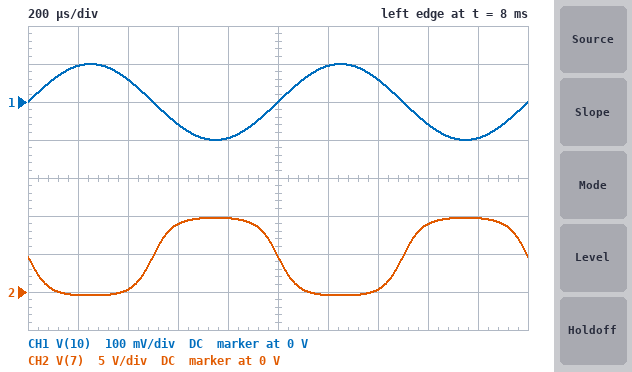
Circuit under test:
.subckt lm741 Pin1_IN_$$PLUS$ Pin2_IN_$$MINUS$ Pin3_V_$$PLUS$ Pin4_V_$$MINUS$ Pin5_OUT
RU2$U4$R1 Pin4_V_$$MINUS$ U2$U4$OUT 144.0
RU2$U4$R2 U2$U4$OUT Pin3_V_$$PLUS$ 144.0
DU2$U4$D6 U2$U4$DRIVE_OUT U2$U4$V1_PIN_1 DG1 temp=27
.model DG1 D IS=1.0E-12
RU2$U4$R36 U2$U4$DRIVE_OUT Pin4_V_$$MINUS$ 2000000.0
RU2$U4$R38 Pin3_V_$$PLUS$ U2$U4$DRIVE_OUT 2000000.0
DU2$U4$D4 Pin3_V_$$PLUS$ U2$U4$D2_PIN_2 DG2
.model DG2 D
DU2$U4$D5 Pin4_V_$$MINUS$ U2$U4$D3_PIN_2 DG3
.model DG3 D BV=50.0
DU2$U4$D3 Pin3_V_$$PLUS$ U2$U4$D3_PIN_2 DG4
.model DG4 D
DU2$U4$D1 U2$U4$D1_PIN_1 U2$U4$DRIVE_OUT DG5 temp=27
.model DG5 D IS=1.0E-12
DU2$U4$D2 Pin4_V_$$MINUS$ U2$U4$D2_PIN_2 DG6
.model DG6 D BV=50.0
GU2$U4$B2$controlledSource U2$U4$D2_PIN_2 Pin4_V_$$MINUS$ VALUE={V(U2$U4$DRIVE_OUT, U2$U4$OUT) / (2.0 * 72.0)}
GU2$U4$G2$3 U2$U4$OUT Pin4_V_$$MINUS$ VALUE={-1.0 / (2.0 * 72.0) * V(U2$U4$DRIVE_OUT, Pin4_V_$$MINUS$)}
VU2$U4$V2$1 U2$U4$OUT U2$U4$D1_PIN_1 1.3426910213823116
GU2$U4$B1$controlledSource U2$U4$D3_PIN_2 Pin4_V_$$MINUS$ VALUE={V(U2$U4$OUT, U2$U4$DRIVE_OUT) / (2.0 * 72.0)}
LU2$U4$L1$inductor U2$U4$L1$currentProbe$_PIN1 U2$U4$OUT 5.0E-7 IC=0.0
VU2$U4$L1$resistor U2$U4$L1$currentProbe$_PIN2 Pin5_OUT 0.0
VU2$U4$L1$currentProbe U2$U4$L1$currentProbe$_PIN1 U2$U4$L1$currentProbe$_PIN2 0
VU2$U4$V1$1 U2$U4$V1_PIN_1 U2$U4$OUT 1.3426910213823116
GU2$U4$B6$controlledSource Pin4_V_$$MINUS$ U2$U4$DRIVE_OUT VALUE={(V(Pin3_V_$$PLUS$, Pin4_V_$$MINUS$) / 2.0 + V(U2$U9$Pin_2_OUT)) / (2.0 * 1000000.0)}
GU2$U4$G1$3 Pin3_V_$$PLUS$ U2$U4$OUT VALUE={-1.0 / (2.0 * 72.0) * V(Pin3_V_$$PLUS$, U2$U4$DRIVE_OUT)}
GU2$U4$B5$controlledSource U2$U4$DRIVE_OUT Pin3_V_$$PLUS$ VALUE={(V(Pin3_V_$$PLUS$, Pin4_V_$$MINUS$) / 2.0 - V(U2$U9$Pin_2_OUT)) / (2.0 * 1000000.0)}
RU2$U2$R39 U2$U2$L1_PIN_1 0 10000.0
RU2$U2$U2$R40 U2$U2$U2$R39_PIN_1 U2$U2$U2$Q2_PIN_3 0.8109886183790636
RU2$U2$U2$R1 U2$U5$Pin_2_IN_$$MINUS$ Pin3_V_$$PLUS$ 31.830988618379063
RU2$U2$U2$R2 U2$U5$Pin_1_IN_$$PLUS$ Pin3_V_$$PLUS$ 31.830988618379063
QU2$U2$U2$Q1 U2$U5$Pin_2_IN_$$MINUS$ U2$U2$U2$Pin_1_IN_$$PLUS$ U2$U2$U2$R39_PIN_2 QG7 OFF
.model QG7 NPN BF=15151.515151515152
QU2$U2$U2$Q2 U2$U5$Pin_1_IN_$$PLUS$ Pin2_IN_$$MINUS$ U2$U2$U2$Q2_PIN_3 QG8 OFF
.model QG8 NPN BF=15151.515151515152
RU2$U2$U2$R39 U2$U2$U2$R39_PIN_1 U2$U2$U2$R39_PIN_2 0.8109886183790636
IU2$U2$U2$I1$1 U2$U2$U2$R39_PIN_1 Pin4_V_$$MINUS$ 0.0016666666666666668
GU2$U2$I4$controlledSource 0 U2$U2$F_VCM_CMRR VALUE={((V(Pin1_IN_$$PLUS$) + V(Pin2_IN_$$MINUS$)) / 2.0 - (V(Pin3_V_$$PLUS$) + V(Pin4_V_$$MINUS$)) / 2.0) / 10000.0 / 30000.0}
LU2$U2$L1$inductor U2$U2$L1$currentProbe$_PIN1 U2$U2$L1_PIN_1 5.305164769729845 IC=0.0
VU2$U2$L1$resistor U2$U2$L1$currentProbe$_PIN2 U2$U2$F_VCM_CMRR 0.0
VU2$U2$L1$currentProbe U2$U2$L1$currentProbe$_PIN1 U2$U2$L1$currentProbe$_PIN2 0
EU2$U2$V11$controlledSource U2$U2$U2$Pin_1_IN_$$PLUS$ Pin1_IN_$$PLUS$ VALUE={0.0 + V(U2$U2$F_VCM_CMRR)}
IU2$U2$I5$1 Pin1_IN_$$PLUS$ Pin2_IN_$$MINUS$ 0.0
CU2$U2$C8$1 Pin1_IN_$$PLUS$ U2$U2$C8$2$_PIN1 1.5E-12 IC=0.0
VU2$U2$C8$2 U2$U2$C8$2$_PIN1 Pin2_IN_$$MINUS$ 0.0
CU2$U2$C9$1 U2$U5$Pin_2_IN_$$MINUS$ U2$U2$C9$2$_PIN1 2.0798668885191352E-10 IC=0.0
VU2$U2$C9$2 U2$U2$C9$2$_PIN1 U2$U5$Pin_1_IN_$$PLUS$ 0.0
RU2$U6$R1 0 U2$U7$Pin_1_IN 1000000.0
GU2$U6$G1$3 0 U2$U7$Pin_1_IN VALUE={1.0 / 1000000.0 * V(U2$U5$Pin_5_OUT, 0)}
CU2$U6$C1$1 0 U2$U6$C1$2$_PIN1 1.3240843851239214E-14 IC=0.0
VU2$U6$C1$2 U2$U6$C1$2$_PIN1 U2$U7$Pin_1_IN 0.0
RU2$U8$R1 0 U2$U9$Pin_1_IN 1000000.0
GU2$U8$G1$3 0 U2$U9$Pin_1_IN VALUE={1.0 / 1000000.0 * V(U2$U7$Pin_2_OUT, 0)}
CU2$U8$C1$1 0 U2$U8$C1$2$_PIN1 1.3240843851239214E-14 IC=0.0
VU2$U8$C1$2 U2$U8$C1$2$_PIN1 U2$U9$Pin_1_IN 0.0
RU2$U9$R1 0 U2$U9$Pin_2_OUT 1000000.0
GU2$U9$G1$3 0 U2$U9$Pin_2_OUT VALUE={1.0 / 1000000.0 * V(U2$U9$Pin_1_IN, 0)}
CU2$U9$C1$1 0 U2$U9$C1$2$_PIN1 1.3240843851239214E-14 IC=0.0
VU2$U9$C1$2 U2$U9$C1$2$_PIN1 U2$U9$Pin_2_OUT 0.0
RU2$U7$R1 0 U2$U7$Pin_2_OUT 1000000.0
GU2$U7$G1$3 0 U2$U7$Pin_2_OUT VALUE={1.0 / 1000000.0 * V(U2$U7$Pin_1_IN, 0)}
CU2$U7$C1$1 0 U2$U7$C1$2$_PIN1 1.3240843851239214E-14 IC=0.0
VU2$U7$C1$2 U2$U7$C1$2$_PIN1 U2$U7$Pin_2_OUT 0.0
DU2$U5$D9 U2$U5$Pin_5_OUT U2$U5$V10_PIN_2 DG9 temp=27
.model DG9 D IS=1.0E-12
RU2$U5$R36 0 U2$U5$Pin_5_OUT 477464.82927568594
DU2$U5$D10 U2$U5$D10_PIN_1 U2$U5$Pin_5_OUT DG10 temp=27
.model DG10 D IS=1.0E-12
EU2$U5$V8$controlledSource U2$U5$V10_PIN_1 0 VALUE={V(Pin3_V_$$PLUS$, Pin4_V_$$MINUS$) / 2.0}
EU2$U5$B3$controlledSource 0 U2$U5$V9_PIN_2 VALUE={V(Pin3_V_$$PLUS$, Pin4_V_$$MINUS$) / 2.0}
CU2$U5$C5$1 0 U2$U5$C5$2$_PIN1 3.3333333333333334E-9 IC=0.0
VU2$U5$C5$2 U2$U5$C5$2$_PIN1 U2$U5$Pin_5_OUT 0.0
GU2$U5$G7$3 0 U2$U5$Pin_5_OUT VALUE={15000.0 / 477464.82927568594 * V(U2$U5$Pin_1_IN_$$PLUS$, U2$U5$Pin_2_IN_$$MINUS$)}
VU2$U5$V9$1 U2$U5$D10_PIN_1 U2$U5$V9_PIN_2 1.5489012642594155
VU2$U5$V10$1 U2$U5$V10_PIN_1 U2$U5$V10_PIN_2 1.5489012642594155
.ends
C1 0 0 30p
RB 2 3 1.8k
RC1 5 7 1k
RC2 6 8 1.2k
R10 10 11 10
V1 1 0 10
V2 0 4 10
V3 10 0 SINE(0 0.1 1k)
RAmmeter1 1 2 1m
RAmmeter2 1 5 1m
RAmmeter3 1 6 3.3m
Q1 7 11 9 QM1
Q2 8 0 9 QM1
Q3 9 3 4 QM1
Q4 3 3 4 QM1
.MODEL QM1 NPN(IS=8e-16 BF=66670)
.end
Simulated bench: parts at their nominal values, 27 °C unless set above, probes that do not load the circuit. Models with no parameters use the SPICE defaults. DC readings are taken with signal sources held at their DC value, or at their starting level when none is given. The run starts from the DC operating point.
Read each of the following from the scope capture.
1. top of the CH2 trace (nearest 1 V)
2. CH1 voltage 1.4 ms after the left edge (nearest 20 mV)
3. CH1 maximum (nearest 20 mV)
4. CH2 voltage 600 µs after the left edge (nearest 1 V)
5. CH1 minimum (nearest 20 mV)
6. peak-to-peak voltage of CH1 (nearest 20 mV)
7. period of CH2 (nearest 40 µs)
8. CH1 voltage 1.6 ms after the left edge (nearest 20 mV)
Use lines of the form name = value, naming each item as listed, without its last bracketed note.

top of the CH2 trace = 10 V
CH1 voltage 1.4 ms after the left edge = 60 mV
CH1 maximum = 100 mV
CH2 voltage 600 µs after the left edge = 9 V
CH1 minimum = -100 mV
peak-to-peak voltage of CH1 = 200 mV
period of CH2 = 1.00 ms
CH1 voltage 1.6 ms after the left edge = -60 mV
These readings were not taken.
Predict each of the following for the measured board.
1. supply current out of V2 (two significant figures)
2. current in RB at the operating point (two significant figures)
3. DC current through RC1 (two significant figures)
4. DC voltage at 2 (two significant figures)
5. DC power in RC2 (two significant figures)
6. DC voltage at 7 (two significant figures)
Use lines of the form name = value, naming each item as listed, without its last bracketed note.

supply current out of V2 = 21 mA
current in RB at the operating point = 11 mA
DC current through RC1 = 5.3 mA
DC voltage at 2 = 10 V
DC power in RC2 = 34 mW
DC voltage at 7 = 4.7 V
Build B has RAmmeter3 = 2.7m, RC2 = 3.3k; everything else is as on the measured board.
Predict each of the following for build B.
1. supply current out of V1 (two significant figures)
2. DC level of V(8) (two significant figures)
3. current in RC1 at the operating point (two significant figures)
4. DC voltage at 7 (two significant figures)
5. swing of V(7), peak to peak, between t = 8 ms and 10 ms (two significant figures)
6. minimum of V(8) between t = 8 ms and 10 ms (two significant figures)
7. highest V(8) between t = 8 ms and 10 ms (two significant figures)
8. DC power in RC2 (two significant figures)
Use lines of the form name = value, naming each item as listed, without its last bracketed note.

supply current out of V1 = 20 mA
DC level of V(8) = -730 mV
current in RC1 at the operating point = 6.0 mA
DC voltage at 7 = 4.0 V
swing of V(7), peak to peak, between t = 8 ms and 10 ms = 10 V
minimum of V(8) between t = 8 ms and 10 ms = -770 mV
highest V(8) between t = 8 ms and 10 ms = 9.3 V
DC power in RC2 = 35 mW
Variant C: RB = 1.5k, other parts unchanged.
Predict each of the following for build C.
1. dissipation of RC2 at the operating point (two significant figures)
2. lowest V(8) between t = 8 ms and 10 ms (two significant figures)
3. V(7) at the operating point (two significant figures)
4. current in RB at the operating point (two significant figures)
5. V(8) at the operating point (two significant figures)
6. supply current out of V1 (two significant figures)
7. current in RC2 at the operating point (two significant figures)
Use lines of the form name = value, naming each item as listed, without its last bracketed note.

dissipation of RC2 at the operating point = 49 mW
lowest V(8) between t = 8 ms and 10 ms = -750 mV
V(7) at the operating point = 3.6 V
current in RB at the operating point = 13 mA
V(8) at the operating point = 2.3 V
supply current out of V1 = 26 mA
current in RC2 at the operating point = 6.4 mA
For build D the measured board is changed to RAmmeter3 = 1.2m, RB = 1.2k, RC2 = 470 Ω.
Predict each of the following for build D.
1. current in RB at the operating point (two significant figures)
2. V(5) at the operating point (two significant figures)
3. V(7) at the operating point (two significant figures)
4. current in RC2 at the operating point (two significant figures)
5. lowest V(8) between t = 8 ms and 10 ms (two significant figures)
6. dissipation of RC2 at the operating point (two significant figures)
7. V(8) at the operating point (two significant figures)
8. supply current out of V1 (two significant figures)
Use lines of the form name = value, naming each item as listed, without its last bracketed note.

current in RB at the operating point = 16 mA
V(5) at the operating point = 10 V
V(7) at the operating point = 2.0 V
current in RC2 at the operating point = 8.0 mA
lowest V(8) between t = 8 ms and 10 ms = 2.6 V
dissipation of RC2 at the operating point = 30 mW
V(8) at the operating point = 6.2 V
supply current out of V1 = 32 mA
